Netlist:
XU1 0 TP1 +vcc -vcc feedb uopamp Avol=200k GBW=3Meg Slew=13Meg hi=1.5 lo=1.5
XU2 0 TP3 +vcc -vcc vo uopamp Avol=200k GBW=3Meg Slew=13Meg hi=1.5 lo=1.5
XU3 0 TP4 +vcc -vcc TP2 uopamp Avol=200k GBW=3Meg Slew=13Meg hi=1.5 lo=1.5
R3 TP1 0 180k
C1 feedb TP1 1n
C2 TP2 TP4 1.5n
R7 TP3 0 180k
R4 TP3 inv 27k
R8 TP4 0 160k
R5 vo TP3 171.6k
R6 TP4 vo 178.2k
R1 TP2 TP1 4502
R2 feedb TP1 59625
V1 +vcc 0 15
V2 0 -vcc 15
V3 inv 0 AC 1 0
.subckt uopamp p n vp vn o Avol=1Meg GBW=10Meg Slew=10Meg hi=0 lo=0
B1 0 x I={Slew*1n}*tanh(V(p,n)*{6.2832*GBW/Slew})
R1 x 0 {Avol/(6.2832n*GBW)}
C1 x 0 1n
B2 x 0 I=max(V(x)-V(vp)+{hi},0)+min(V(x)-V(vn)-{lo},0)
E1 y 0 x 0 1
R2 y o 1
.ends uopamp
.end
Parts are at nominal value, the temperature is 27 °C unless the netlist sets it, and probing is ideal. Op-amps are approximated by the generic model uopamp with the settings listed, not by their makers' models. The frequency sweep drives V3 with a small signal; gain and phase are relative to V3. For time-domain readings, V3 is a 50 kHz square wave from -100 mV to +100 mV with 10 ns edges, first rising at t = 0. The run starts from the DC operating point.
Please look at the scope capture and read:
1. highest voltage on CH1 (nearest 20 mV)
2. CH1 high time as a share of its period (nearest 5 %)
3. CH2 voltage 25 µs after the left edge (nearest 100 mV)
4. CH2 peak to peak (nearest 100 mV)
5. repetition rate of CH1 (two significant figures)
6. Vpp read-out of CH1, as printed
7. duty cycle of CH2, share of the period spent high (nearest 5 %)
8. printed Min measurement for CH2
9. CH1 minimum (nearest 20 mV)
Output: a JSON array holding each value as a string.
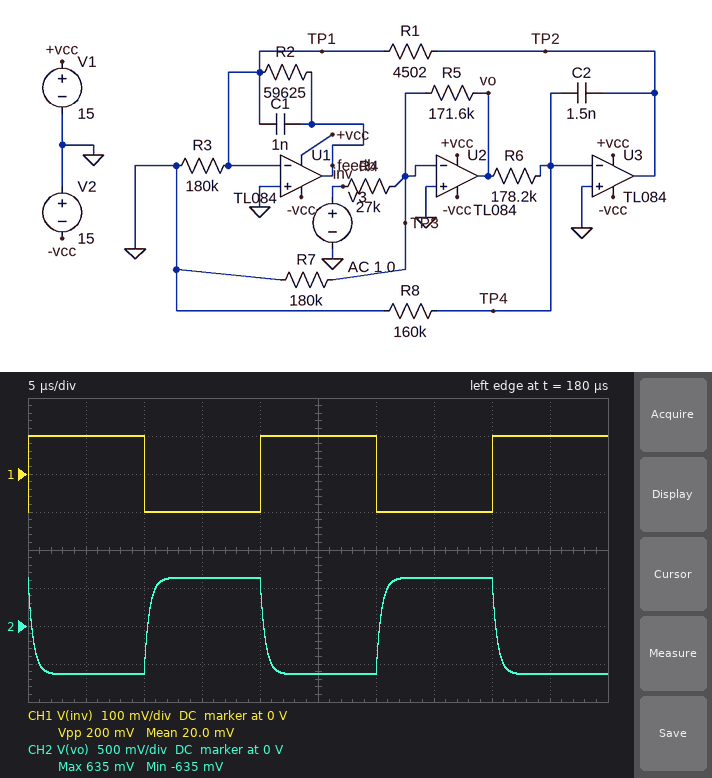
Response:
["100 mV", "50 %", "-600 mV", "1.3 V", "50 kHz", "200 mV", "50 %", "-635 mV", "-100 mV"]
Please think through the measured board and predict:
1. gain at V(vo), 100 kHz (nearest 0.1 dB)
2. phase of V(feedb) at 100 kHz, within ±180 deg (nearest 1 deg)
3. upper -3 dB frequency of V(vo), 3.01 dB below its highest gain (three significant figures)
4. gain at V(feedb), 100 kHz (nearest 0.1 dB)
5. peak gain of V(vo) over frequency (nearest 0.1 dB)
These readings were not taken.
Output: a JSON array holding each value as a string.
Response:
["15.7 dB", "-18 deg", "361 kHz", "-37.9 dB", "16.1 dB"]
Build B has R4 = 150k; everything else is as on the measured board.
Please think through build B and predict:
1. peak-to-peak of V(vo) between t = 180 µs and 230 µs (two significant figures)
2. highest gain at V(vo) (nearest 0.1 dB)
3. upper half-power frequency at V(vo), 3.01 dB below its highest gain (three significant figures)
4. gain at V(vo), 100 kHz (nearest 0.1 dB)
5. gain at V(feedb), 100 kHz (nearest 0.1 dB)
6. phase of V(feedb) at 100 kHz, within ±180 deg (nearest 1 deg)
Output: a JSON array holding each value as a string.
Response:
["230 mV", "1.2 dB", "969 kHz", "1.1 dB", "-52.5 dB", "-8 deg"]
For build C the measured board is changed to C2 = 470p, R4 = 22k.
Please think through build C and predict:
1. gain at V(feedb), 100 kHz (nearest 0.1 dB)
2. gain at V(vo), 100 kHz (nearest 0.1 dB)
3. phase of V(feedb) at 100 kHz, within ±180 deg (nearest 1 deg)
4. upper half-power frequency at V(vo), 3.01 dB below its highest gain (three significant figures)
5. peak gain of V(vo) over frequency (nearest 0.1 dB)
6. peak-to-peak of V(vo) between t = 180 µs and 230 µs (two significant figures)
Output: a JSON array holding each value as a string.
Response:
["-26.2 dB", "17.4 dB", "-20 deg", "308 kHz", "17.8 dB", "1.6 V"]
